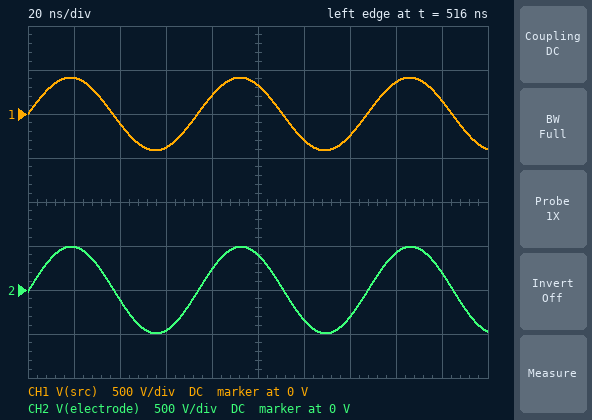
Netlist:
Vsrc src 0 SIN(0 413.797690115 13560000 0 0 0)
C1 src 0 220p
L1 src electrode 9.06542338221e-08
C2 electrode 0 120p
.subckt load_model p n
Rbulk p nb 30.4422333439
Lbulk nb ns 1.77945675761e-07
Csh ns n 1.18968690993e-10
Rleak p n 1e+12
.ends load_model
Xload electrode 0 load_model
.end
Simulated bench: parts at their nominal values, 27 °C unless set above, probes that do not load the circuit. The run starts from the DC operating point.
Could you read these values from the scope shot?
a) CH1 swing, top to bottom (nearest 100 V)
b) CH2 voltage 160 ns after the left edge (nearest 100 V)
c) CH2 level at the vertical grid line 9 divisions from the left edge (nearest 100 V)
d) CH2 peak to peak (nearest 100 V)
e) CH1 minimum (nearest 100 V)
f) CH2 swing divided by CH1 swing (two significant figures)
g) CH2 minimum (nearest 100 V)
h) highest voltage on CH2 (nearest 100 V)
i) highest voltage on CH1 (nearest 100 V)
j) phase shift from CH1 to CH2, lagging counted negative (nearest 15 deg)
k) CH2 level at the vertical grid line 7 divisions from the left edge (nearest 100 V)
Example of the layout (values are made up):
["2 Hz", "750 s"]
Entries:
["800 V", "400 V", "200 V", "1.0 kV", "-400 V", "1.2", "-500 V", "500 V", "400 V", "0 deg", "-300 V"]
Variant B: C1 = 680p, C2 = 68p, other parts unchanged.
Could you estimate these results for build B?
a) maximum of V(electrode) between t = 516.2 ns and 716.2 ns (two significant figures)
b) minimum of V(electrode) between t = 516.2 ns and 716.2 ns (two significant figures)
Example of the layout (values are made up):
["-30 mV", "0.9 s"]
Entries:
["470 V", "-470 V"]
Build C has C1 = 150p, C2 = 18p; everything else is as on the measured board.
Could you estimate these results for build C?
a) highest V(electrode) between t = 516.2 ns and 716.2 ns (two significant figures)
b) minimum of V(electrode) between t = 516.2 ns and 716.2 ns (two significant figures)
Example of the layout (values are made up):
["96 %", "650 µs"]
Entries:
["460 V", "-460 V"]
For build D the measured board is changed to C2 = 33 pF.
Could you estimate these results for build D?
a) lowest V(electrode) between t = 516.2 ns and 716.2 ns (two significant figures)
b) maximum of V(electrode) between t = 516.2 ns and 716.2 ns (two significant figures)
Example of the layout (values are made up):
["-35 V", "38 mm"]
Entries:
["-460 V", "460 V"]
